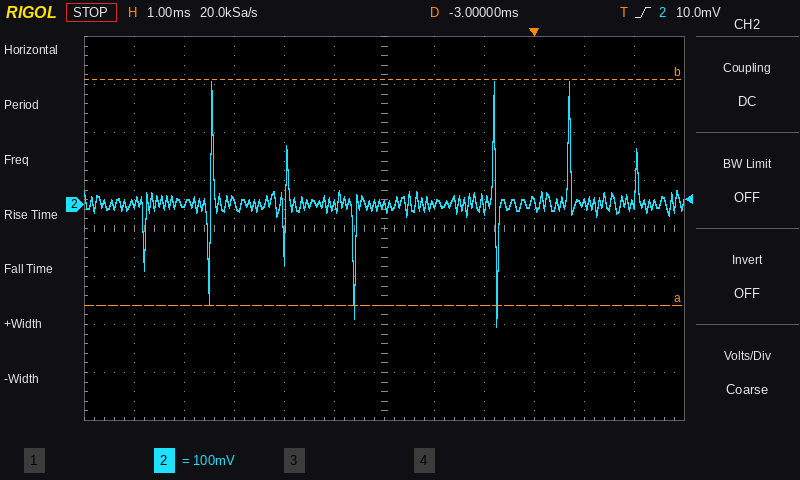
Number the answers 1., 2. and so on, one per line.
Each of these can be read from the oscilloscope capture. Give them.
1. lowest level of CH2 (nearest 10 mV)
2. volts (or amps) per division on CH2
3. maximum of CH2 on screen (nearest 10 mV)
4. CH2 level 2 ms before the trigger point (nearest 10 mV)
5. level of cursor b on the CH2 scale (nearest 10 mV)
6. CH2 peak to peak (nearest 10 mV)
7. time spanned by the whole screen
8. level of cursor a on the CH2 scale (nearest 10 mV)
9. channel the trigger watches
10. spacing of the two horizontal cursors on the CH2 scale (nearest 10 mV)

1. -250 mV
2. 100 mV
3. 260 mV
4. 0 mV
5. 260 mV
6. 510 mV
7. 12 ms
8. -210 mV
9. CH2
10. 470 mV
